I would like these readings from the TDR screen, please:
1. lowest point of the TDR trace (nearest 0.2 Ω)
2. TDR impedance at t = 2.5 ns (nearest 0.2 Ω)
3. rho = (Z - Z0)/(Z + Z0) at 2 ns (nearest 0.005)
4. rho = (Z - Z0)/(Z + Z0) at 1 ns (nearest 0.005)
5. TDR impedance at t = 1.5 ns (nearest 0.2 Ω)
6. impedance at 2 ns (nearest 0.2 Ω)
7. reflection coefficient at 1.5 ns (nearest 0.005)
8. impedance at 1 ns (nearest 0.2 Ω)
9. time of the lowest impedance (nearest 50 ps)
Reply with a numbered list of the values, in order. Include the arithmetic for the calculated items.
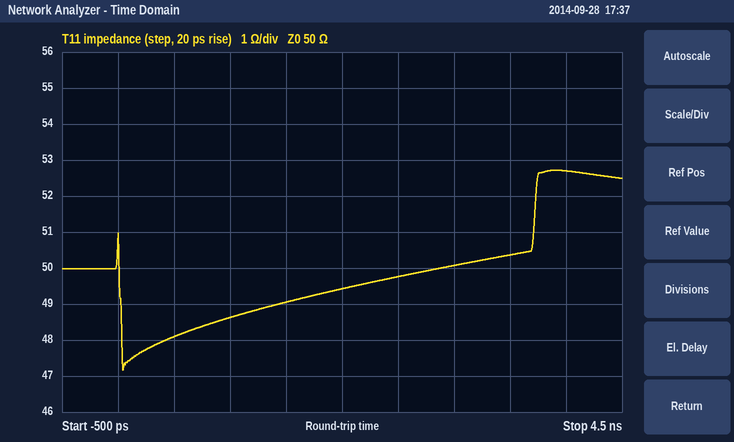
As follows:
1. 47.2 Ω
2. 49.8 Ω
3. (49.4 − 50)/(49.4 + 50) ≈ -0.00604, so -0.005 to the nearest 0.005
4. (48.6 − 50)/(48.6 + 50) ≈ -0.0142, so -0.015 to the nearest 0.005
5. 49.0 Ω
6. 49.4 Ω
7. (49 − 50)/(49 + 50) ≈ -0.010
8. 48.6 Ω
9. 50 ps
